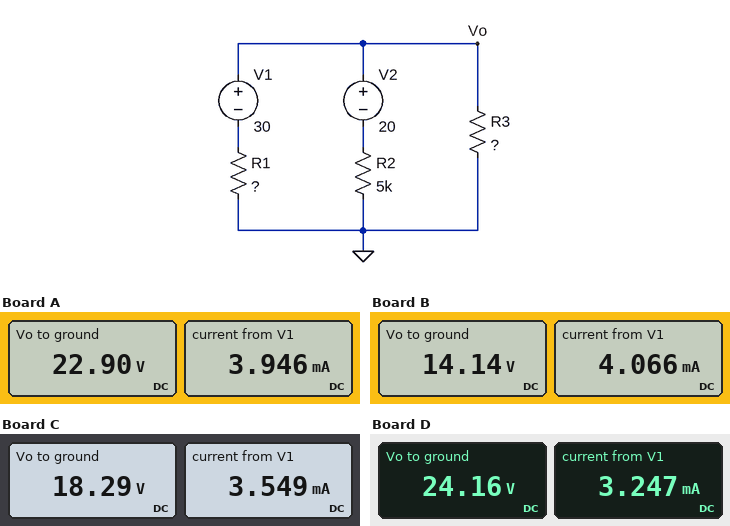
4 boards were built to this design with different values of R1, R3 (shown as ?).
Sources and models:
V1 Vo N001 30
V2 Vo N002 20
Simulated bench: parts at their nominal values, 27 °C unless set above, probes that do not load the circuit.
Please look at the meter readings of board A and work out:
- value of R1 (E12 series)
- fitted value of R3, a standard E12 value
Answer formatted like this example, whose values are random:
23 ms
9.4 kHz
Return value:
1.8 kΩ
6.8 kΩ
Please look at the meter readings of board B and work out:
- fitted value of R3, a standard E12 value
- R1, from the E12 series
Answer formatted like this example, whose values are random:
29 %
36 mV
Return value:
2.7 kΩ
3.9 kΩ
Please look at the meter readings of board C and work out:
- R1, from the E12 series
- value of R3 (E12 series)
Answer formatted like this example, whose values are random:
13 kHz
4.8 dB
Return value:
3.3 kΩ
4.7 kΩ
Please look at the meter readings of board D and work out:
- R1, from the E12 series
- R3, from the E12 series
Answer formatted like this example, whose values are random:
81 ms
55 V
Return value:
1.8 kΩ
10 kΩ
